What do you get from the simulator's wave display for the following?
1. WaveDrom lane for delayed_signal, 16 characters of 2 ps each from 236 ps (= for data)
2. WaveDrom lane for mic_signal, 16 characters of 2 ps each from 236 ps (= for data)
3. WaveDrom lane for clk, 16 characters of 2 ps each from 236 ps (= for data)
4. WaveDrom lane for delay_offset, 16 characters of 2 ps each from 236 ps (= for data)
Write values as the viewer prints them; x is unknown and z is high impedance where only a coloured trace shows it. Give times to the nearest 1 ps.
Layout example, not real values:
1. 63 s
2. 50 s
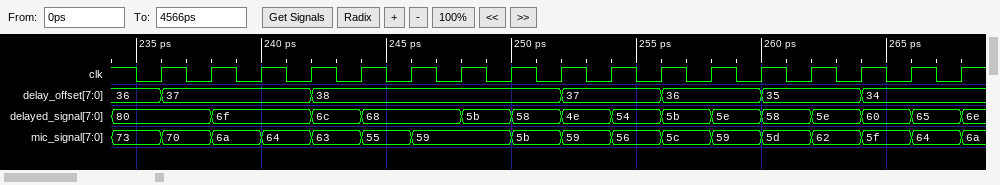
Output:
1. {name: 'delayed_signal', wave: '==.==.==========', data: '80 6f 6c 68 5b 58 4e 54 5b 5e 58 5e 60 65'}
2. {name: 'mic_signal', wave: '======.=========', data: '70 6a 64 63 55 59 5b 59 56 5c 59 5d 62 5f 64'}
3. {name: 'clk', wave: 'p...............'}
4. {name: 'delay_offset', wave: '=..=....=.=.=.=.', data: '37 38 37 36 35 34'}
